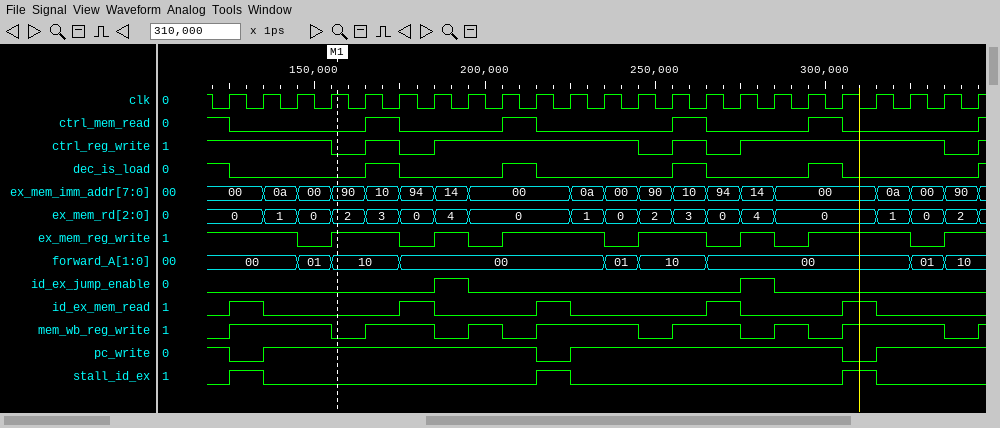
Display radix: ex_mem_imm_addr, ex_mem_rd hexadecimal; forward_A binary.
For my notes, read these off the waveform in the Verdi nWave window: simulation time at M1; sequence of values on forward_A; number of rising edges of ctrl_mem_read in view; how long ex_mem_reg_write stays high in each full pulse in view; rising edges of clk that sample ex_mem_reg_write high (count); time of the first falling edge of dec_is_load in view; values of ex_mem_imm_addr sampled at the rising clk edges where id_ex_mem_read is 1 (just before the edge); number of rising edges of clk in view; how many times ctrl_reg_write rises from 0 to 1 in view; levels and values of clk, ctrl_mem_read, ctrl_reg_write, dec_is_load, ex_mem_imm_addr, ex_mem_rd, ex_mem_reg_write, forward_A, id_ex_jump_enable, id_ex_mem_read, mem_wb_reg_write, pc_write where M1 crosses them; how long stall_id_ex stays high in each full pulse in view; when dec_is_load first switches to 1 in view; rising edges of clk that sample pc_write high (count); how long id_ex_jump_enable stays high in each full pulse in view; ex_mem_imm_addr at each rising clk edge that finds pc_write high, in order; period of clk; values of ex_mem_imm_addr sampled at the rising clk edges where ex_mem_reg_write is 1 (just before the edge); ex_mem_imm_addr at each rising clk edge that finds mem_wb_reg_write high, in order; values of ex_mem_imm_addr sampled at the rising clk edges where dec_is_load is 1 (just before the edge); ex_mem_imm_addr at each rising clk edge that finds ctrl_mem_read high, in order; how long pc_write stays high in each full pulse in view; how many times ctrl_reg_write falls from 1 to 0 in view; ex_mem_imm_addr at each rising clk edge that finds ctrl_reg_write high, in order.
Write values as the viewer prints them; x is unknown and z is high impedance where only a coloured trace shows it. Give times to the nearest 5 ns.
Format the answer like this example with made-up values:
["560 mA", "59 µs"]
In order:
["155 ns", "00, 01, 10, 00, 01, 10, 00, 01, 10", "5", "20 ns, 10 ns, 30 ns, 20 ns, 10 ns, 30 ns", "16", "125 ns", "00, 94, 00, 94, 00", "23", "5", "clk=1, ctrl_mem_read=0, ctrl_reg_write=0, dec_is_load=0, ex_mem_imm_addr=90, ex_mem_rd=2, ex_mem_reg_write=1, forward_A=10, id_ex_jump_enable=0, id_ex_mem_read=0, mem_wb_reg_write=0, pc_write=1", "10 ns, 10 ns, 10 ns", "165 ns", "20", "10 ns, 10 ns", "00, 0a, 00, 90, 10, 94, 14, 00, 00, 0a, 00, 90, 10, 94, 14, 00, 00, 0a, 00, 90", "10 ns", "00, 00, 0a, 90, 10, 14, 00, 00, 0a, 90, 10, 14, 00, 00, 0a, 90", "00, 0a, 00, 10, 94, 00, 00, 0a, 00, 10, 94, 00, 00, 0a, 00", "00, 10, 00, 10, 00", "00, 10, 00, 10, 00", "80 ns, 80 ns", "5", "00, 00, 0a, 00, 10, 14, 00, 00, 00, 0a, 00, 10, 14, 00, 00, 00, 0a, 00"]
